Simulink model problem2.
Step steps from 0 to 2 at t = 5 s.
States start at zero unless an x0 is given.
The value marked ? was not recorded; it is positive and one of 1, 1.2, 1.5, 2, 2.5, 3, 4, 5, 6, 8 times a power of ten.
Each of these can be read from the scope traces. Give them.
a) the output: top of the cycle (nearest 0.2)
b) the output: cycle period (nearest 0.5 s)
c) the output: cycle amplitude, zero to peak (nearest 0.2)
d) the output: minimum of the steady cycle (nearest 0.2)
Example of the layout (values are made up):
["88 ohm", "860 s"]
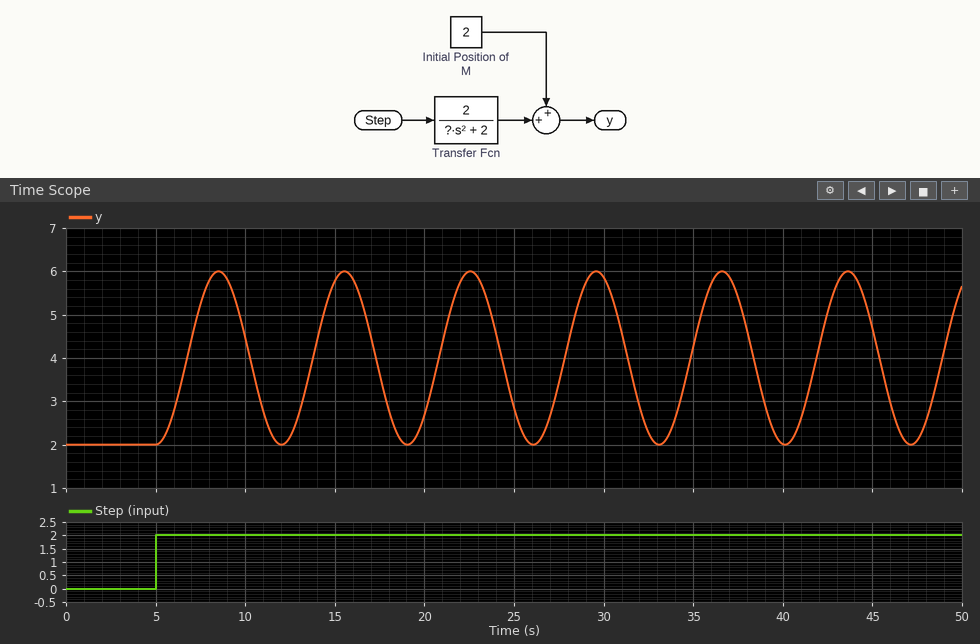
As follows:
["6.0", "7.0 s", "2.0", "2.0"]
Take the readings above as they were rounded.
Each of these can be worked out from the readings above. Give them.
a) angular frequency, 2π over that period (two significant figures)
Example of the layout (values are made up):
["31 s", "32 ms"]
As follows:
["0.90 rad/s"]
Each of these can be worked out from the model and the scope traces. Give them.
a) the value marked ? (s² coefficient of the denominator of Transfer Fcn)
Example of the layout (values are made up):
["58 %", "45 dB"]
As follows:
["2.5"]
